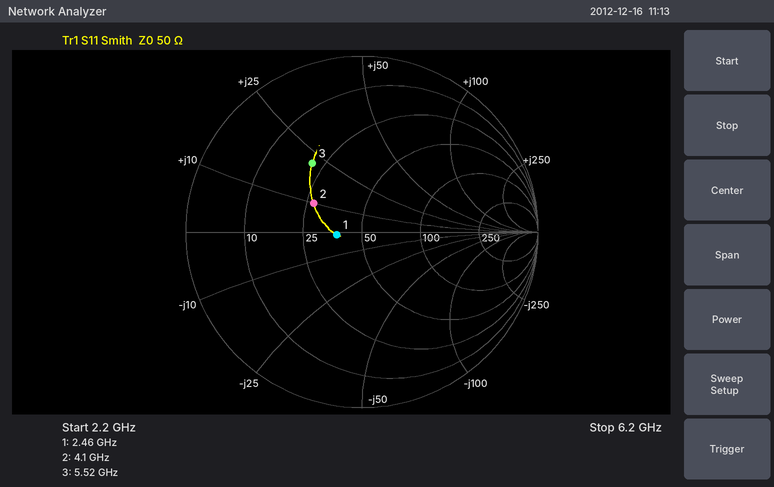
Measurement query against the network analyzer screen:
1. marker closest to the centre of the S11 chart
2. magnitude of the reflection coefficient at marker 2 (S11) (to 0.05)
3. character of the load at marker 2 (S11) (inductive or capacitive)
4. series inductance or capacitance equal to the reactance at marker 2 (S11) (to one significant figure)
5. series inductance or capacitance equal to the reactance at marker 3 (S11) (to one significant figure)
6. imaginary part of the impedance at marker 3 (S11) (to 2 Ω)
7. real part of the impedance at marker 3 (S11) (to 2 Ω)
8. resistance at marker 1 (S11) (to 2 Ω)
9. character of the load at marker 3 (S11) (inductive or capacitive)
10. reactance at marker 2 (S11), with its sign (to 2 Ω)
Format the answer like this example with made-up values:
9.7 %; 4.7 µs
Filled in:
marker 1; 0.30; inductive; 400 pH; 600 pH; +22 Ω; 22 Ω; 38 Ω; inductive; +10 Ω
